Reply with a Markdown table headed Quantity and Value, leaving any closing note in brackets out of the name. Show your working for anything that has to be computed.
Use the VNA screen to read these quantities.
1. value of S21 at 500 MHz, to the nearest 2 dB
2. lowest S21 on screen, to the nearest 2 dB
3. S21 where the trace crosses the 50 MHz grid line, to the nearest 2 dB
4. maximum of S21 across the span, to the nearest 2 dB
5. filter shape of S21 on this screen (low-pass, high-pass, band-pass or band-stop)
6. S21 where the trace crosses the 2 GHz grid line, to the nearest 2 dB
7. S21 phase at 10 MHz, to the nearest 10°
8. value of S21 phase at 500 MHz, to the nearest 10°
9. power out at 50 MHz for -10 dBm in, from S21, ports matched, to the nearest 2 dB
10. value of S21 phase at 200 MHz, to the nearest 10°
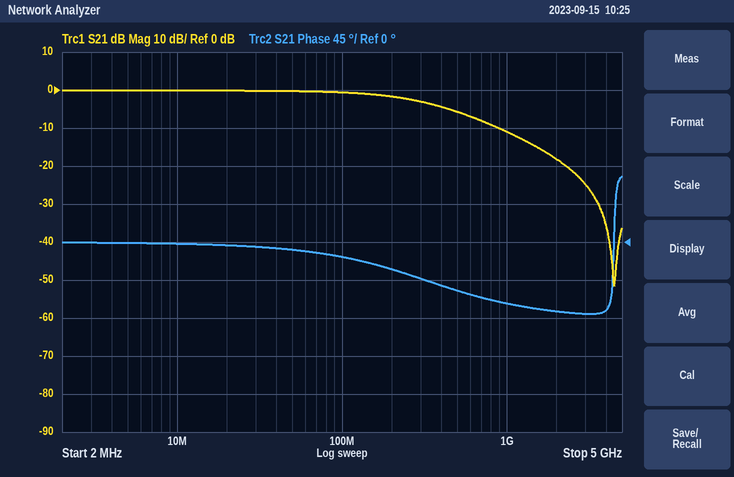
| Quantity | Value |
|---|---|
| value of S21 at 500 MHz, to the nearest 2 dB | -6 dB |
| lowest S21 on screen, to the nearest 2 dB | -52 dB |
| S21 where the trace crosses the 50 MHz grid line, to the nearest 2 dB | 0 dB |
| maximum of S21 across the span, to the nearest 2 dB | 0 dB |
| filter shape of S21 on this screen | low-pass |
| S21 where the trace crosses the 2 GHz grid line, to the nearest 2 dB | -18 dB |
| S21 phase at 10 MHz, to the nearest 10° | 0° |
| value of S21 phase at 500 MHz, to the nearest 10° | -60° |
| power out at 50 MHz for -10 dBm in, from S21, ports matched, to the nearest 2 dB | -10 dBm + (0 dB) = -10 dBm |
| value of S21 phase at 200 MHz, to the nearest 10° | -30° |
